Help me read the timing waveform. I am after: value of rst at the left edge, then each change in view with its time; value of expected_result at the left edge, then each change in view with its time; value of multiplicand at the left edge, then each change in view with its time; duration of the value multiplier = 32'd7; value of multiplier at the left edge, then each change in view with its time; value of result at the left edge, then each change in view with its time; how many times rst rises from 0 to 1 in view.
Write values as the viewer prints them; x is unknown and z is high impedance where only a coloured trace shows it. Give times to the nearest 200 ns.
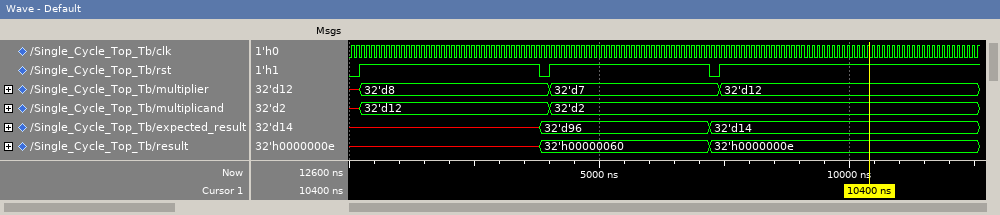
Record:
0, 1 at 200 ns, 0 at 3800 ns, 1 at 4000 ns, 0 at 7200 ns, 1 at 7400 ns
x, 32'd96 at 3800 ns, 32'd14 at 7200 ns
x, 32'd12 at 200 ns, 32'd2 at 4000 ns
3400 ns
x, 32'd8 at 200 ns, 32'd7 at 4000 ns, 32'd12 at 7400 ns
x, 32'h00000060 at 3800 ns, 32'h0000000e at 7200 ns
3
